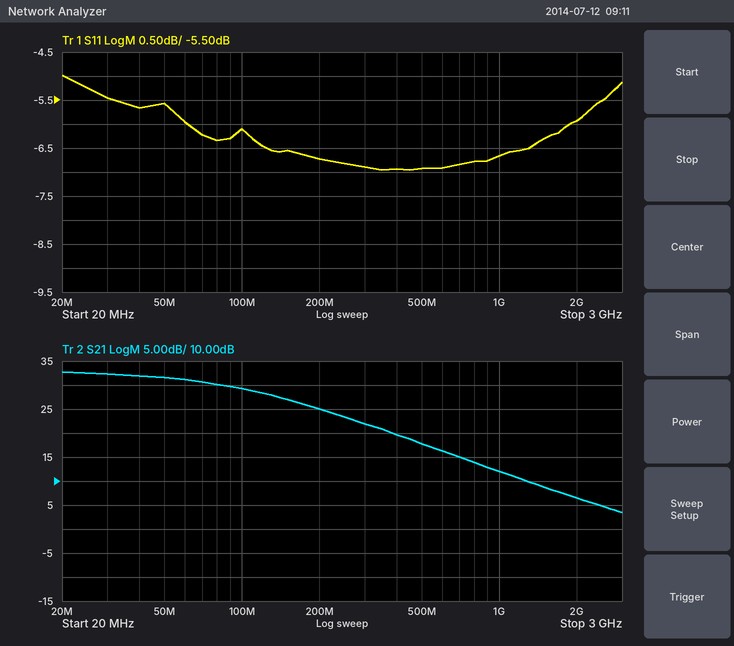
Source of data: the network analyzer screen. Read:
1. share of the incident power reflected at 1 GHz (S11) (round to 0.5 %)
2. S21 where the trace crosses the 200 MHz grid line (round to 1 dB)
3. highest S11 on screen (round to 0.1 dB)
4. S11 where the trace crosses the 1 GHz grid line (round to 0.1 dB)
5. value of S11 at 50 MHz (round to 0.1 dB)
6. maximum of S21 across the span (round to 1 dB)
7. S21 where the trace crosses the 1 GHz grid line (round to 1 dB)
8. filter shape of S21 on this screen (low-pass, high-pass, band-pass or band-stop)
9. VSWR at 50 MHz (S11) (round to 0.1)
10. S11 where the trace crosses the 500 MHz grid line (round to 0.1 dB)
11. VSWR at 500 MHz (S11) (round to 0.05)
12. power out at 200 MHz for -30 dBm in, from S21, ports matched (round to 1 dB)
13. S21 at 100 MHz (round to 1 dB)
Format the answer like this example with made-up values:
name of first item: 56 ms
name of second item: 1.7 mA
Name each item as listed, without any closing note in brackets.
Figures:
share of the incident power reflected at 1 GHz (S11): 21.5 %
S21 where the trace crosses the 200 MHz grid line: 25 dB
highest S11 on screen: -5.0 dB
S11 where the trace crosses the 1 GHz grid line: -6.7 dB
value of S11 at 50 MHz: -5.6 dB
maximum of S21 across the span: 33 dB
S21 where the trace crosses the 1 GHz grid line: 12 dB
filter shape of S21 on this screen: low-pass
VSWR at 50 MHz (S11): 3.2
S11 where the trace crosses the 500 MHz grid line: -6.9 dB
VSWR at 500 MHz (S11): 2.65
power out at 200 MHz for -30 dBm in, from S21, ports matched: -5 dBm
S21 at 100 MHz: 29 dB
